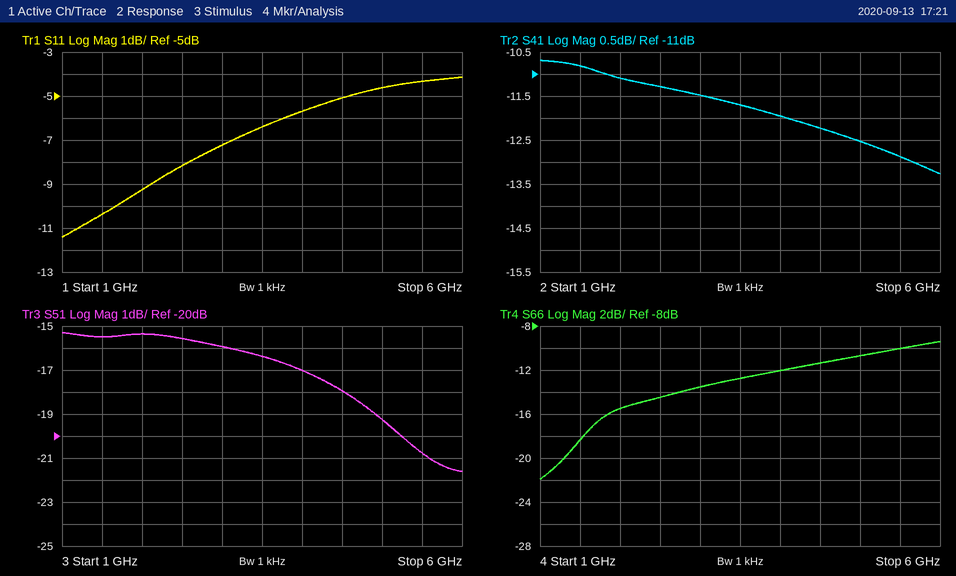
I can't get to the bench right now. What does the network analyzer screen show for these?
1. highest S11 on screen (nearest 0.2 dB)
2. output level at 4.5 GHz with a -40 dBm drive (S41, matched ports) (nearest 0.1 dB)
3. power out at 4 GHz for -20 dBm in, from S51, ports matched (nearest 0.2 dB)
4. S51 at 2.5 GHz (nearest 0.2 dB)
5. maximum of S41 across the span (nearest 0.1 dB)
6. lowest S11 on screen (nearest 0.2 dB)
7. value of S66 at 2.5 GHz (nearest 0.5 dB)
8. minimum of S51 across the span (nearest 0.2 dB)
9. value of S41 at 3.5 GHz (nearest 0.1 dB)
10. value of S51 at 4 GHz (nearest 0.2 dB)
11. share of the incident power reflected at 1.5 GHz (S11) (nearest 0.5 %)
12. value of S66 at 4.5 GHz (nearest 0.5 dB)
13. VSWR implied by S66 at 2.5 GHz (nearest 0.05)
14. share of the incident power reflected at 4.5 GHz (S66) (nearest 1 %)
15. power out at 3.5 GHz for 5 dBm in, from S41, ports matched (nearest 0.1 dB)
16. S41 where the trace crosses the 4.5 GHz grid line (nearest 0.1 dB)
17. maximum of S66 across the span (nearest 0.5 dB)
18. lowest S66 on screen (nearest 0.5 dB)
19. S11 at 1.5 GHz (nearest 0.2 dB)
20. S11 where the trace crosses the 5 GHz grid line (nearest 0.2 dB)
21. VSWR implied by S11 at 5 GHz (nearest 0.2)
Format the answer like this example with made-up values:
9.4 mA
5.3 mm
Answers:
-4.2 dB
-52.2 dBm
-37.0 dBm
-15.6 dB
-10.7 dB
-11.4 dB
-14.5 dB
-21.6 dB
-11.7 dB
-17.0 dB
9.0 %
-11.5 dB
1.45
7 %
-6.7 dBm
-12.2 dB
-9.5 dB
-22.0 dB
-10.4 dB
-4.6 dB
3.8
